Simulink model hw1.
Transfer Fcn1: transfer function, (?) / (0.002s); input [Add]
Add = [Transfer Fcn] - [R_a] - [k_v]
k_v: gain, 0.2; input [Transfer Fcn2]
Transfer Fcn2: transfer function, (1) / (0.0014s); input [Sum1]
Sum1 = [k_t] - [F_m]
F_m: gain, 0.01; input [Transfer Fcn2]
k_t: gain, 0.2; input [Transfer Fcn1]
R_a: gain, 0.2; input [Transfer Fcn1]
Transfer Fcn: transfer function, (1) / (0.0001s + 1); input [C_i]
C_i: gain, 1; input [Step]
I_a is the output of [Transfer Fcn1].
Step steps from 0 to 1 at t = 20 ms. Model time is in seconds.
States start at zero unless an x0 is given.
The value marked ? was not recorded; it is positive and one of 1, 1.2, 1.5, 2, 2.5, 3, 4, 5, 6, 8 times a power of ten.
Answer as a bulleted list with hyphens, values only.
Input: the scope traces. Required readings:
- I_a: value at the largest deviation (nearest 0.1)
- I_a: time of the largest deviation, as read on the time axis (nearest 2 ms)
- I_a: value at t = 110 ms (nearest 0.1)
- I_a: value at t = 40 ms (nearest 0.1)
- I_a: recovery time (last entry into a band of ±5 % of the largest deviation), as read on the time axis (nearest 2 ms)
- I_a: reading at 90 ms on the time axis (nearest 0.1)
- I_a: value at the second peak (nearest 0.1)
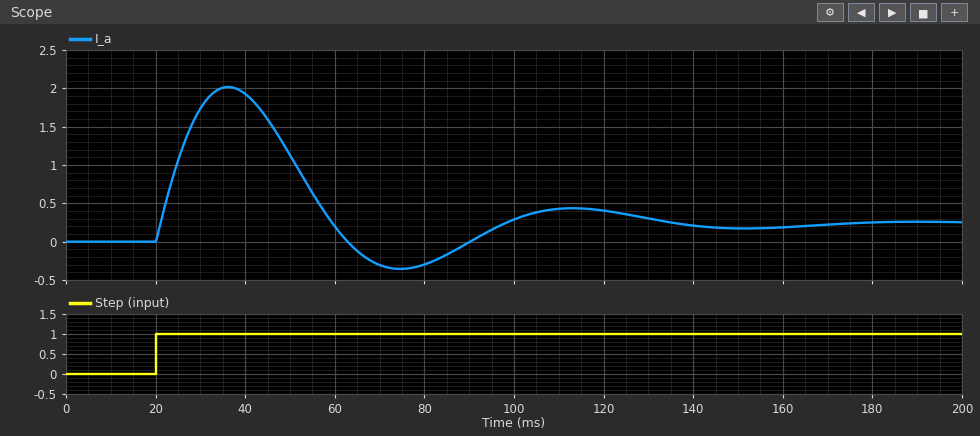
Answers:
- 2.0
- 36 ms
- 0.4
- 1.9
- 126 ms
- 0.0
- 0.4
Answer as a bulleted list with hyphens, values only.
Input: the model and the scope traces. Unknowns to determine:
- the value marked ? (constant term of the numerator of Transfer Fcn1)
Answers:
- 0.5
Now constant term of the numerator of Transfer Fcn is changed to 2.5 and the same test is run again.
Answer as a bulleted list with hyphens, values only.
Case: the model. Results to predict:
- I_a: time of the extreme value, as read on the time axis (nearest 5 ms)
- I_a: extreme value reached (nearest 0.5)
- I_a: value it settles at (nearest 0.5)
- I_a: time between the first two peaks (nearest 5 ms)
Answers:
- 35 ms
- 5.0
- 0.5
- 75 ms
